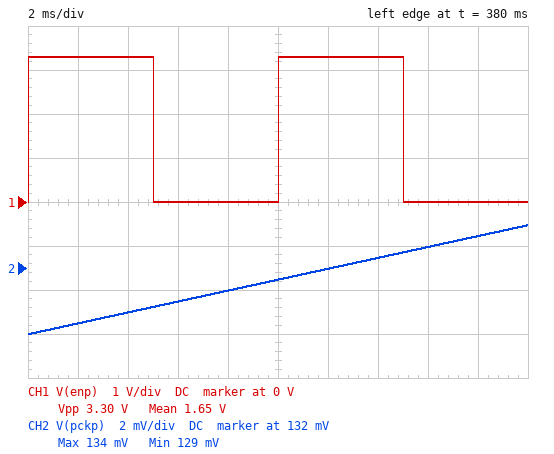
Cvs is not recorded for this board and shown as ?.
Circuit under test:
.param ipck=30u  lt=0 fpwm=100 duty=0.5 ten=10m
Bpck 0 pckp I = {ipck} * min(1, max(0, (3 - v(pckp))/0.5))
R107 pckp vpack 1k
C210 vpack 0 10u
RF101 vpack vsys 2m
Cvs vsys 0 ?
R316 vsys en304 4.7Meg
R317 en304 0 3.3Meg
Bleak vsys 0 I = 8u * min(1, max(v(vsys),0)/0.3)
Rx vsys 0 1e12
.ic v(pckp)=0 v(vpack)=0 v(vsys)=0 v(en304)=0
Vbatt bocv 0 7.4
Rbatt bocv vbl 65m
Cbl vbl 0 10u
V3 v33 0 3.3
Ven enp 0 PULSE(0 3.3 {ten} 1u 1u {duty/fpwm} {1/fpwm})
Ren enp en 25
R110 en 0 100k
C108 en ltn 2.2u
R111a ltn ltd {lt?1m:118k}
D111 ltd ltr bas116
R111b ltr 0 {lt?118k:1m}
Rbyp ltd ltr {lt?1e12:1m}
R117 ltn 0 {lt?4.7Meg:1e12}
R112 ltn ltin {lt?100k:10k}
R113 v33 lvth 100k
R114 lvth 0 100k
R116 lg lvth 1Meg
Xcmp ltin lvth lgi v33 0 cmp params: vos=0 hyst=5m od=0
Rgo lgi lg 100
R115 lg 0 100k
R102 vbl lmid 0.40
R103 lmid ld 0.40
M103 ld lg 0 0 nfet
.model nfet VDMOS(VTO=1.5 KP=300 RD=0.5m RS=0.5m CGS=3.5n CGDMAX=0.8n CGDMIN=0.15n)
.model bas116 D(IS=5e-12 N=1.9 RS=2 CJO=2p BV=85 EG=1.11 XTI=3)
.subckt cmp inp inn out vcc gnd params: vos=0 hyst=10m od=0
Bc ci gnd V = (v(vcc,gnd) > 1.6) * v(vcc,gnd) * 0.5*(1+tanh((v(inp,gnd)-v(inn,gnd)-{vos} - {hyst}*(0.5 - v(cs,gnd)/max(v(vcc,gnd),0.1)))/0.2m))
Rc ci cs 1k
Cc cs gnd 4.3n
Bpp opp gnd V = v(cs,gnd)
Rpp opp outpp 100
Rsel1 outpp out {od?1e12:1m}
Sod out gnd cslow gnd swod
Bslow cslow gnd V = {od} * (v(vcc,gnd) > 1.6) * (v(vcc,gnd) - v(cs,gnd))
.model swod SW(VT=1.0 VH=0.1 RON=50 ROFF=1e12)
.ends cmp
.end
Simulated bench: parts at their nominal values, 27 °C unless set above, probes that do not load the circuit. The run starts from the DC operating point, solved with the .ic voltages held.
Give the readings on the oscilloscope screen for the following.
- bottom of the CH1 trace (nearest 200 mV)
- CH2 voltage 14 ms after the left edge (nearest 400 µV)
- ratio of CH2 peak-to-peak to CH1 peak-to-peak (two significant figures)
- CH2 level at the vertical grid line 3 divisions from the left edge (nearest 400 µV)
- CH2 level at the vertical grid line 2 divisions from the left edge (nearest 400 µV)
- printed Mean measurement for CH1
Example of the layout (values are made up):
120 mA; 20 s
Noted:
0 V; 132.4 mV; 0.0015; 130.4 mV; 130.0 mV; 1.65 V
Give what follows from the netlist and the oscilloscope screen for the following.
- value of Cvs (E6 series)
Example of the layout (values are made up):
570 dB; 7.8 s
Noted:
100 µF
